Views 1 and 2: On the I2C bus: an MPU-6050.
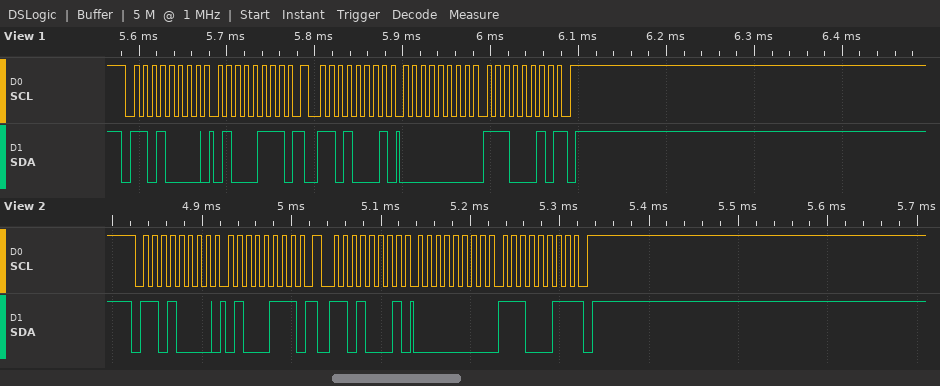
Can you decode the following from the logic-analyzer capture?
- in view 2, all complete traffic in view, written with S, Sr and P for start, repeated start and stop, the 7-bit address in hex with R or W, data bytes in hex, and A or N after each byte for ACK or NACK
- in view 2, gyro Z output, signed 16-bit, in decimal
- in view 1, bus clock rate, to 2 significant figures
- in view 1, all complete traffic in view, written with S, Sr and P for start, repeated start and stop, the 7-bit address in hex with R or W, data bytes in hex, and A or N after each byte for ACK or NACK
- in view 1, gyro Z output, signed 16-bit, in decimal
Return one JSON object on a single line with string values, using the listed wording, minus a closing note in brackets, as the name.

{"in view 2, all complete traffic in view, written with S, Sr and P for start, repeated start and stop, the 7-bit address in hex with R or W, data bytes in hex, and A or N after each byte for ACK or NACK": "S 68W A 47 A Sr 68R A 00 A E3 N P", "in view 2, gyro Z output, signed 16-bit, in decimal": "227", "in view 1, bus clock rate, to 2 significant figures": "100 kHz", "in view 1, all complete traffic in view, written with S, Sr and P for start, repeated start and stop, the 7-bit address in hex with R or W, data bytes in hex, and A or N after each byte for ACK or NACK": "S 68W A 47 A Sr 68R A 00 A E2 N P", "in view 1, gyro Z output, signed 16-bit, in decimal": "226"}
